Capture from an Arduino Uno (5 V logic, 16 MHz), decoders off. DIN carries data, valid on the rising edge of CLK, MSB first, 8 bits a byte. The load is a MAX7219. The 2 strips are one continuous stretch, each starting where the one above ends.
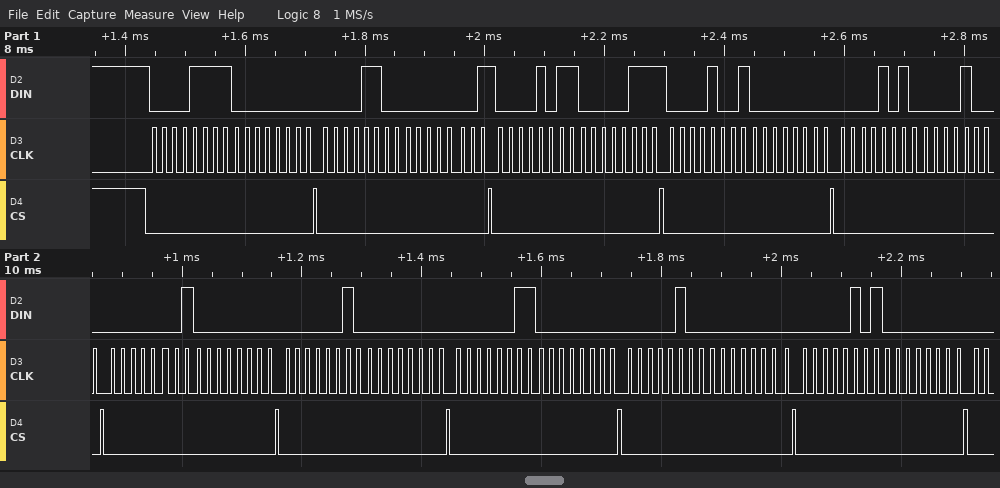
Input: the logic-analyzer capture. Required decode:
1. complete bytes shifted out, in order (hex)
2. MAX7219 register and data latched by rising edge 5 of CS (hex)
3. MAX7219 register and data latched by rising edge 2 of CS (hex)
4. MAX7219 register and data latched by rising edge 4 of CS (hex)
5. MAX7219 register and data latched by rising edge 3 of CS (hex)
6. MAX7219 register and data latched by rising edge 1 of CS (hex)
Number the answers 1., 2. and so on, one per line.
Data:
1. 0F 00 0C 01 0B 07 09 00 0A 08 01 00 02 00 03 00 04 00 05 00
2. register 0xA, data 0x08
3. register 0xC, data 0x01
4. register 0x9, data 0x00
5. register 0xB, data 0x07
6. register 0xF, data 0x00
